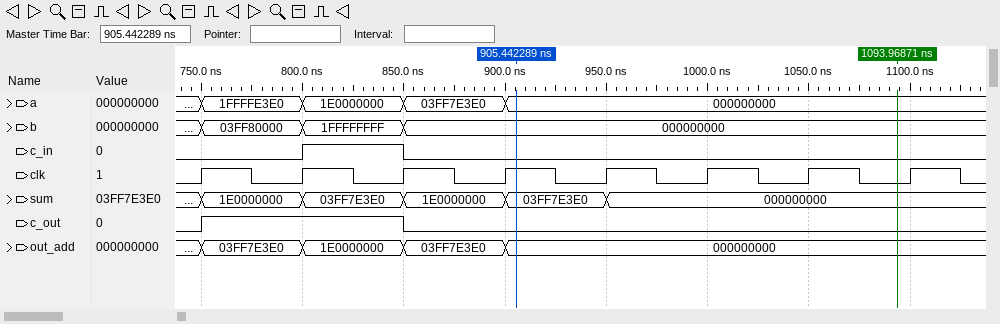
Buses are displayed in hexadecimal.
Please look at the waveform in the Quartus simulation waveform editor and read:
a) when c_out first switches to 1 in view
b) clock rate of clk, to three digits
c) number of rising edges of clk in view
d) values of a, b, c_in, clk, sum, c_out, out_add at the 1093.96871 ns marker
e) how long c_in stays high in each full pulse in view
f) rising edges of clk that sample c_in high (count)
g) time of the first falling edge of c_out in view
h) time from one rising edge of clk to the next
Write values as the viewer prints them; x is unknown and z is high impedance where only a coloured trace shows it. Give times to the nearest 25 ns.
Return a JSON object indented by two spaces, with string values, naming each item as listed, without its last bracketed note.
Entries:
{
  "when c_out first switches to 1 in view": "750 ns",
  "clock rate of clk, to three digits": "20.0 MHz",
  "number of rising edges of clk in view": "8",
  "values of a, b, c_in, clk, sum, c_out, out_add at the 1093.96871 ns marker": "a=000000000, b=000000000, c_in=0, clk=0, sum=000000000, c_out=0, out_add=000000000",
  "how long c_in stays high in each full pulse in view": "50 ns",
  "rising edges of clk that sample c_in high": "1",
  "time of the first falling edge of c_out in view": "850 ns",
  "time from one rising edge of clk to the next": "50 ns"
}
